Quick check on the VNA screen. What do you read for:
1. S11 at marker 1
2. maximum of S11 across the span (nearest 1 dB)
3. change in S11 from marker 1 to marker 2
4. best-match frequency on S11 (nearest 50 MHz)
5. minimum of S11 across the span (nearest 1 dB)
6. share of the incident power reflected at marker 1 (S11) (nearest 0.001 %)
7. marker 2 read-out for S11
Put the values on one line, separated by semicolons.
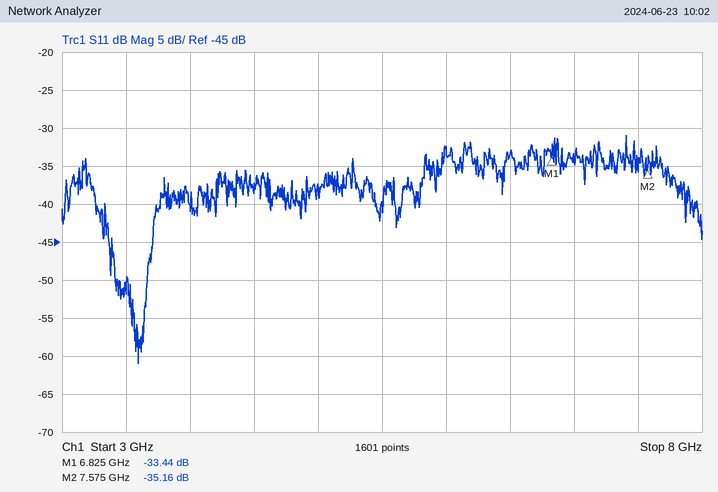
-33.44 dB; -31 dB; -1.72 dB; 3.60 GHz; -61 dB; 0.045 %; -35.16 dB
